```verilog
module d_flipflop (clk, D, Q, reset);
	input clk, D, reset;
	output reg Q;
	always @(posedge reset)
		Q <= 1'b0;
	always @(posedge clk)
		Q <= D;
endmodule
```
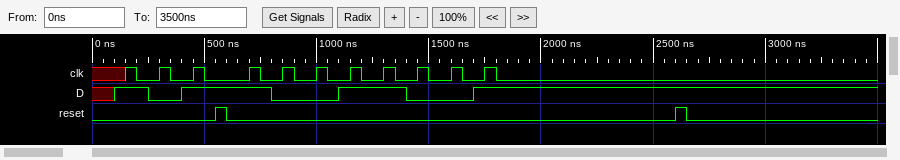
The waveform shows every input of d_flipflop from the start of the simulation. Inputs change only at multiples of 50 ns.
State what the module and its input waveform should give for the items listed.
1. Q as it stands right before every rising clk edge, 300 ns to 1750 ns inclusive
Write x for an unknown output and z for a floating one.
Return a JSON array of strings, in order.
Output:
["1 0 0 1 0 0 1 1 0 0"]
